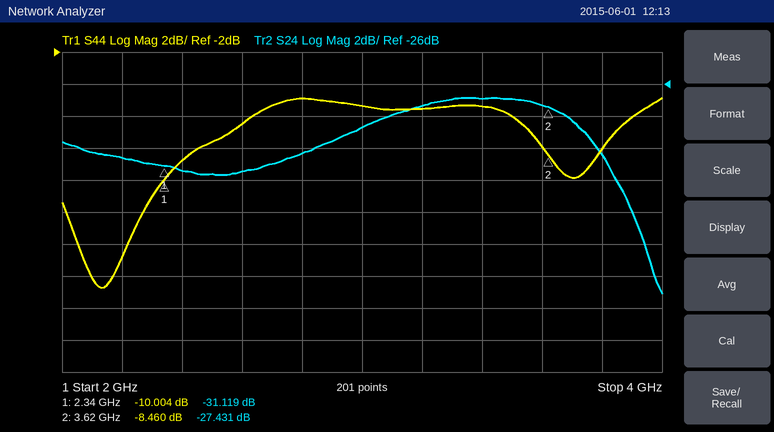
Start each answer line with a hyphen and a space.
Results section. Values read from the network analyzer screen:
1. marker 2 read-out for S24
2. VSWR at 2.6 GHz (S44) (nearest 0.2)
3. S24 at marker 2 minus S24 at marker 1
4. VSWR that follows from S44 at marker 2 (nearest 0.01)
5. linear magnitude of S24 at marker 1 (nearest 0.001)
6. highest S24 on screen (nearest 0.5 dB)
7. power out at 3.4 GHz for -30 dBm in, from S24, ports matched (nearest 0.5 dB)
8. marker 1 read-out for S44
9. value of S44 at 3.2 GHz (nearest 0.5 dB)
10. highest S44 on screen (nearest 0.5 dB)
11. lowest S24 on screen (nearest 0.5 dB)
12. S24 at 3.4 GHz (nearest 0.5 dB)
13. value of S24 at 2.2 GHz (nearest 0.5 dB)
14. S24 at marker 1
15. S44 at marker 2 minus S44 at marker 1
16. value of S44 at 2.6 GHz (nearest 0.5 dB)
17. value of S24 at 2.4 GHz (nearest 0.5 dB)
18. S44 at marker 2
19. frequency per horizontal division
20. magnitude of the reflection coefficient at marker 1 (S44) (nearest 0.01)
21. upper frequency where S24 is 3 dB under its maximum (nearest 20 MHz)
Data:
- -27.431 dB
- 2.8
- 3.688 dB
- 2.21
- 0.028
- -27.0 dB
- -57.0 dBm
- -10.004 dB
- -5.5 dB
- -5.0 dB
- -39.0 dB
- -27.0 dB
- -30.5 dB
- -31.119 dB
- 1.544 dB
- -6.5 dB
- -31.5 dB
- -8.460 dB
- 200 MHz
- 0.32
- 3.78 GHz
